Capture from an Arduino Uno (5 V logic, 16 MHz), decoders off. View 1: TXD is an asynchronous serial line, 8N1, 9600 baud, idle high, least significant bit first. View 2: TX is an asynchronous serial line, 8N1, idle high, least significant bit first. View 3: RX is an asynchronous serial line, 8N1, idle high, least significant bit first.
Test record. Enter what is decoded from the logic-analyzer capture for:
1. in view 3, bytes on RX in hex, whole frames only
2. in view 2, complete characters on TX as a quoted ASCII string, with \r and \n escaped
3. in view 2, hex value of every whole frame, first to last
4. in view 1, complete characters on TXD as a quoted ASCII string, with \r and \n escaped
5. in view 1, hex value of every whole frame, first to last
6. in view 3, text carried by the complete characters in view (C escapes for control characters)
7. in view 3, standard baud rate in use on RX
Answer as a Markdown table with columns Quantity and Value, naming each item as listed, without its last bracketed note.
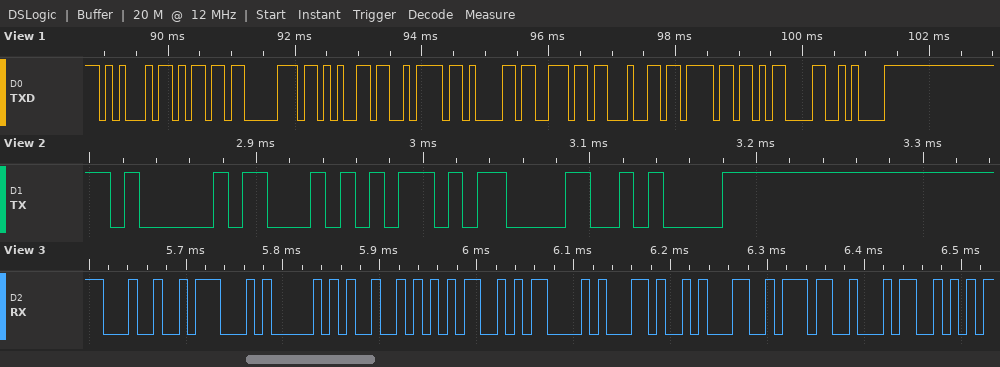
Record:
| Quantity | Value |
|---|---|
| in view 3, bytes on RX in hex, whole frames only | 24 47 50 52 4D 43 2C 31 37 34 |
| in view 2, complete characters on TX as a quoted ASCII string, with \r and \n escaped | "AT\r\n" |
| in view 2, hex value of every whole frame, first to last | 0x41 0x54 0x0D 0x0A |
| in view 1, complete characters on TXD as a quoted ASCII string, with \r and \n escaped | "Empezando\r\n" |
| in view 1, hex value of every whole frame, first to last | 0x45 0x6D 0x70 0x65 0x7A 0x61 0x6E 0x64 0x6F 0x0D 0x0A |
| in view 3, text carried by the complete characters in view | "$GPRMC,174" |
| in view 3, standard baud rate in use on RX | 115200 baud |
